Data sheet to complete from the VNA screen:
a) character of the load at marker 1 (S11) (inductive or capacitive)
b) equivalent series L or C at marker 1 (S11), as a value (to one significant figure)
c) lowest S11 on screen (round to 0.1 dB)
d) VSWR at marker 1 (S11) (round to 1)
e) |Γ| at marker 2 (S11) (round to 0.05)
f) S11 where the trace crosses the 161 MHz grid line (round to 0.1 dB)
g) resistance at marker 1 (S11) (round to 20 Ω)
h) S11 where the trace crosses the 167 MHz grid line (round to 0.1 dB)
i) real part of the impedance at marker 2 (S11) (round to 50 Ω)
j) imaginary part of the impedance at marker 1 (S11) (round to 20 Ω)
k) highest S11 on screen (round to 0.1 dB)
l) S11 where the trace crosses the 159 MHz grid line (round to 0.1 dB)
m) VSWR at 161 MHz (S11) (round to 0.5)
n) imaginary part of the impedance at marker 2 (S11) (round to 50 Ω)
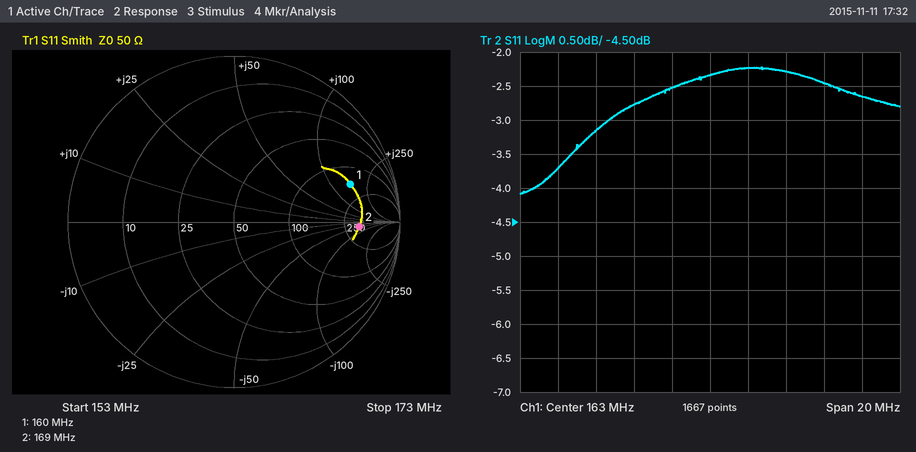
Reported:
inductive
200 nH
-4.1 dB
7
0.75
-2.5 dB
160 Ω
-2.3 dB
350 Ω
+160 Ω
-2.2 dB
-2.8 dB
7.0
-50 Ω
